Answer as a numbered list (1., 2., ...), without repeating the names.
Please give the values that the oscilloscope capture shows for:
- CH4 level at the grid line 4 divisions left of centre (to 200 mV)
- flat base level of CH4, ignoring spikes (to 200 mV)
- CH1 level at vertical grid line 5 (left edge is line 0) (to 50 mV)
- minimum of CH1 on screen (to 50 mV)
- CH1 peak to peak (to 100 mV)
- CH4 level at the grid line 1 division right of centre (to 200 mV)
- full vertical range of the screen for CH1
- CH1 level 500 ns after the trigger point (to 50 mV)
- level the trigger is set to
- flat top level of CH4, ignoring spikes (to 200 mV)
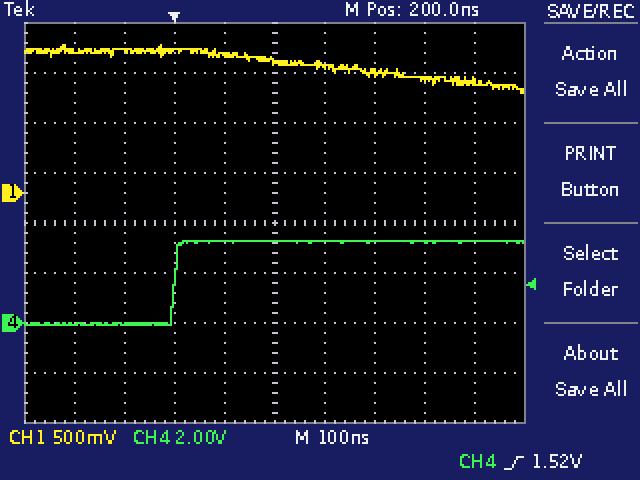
1. 0.0 V
2. 0.0 V
3. 1.30 V
4. 1.00 V
5. 500 mV
6. 3.2 V
7. 4 V
8. 1.15 V
9. 1.52 V
10. 3.2 V
